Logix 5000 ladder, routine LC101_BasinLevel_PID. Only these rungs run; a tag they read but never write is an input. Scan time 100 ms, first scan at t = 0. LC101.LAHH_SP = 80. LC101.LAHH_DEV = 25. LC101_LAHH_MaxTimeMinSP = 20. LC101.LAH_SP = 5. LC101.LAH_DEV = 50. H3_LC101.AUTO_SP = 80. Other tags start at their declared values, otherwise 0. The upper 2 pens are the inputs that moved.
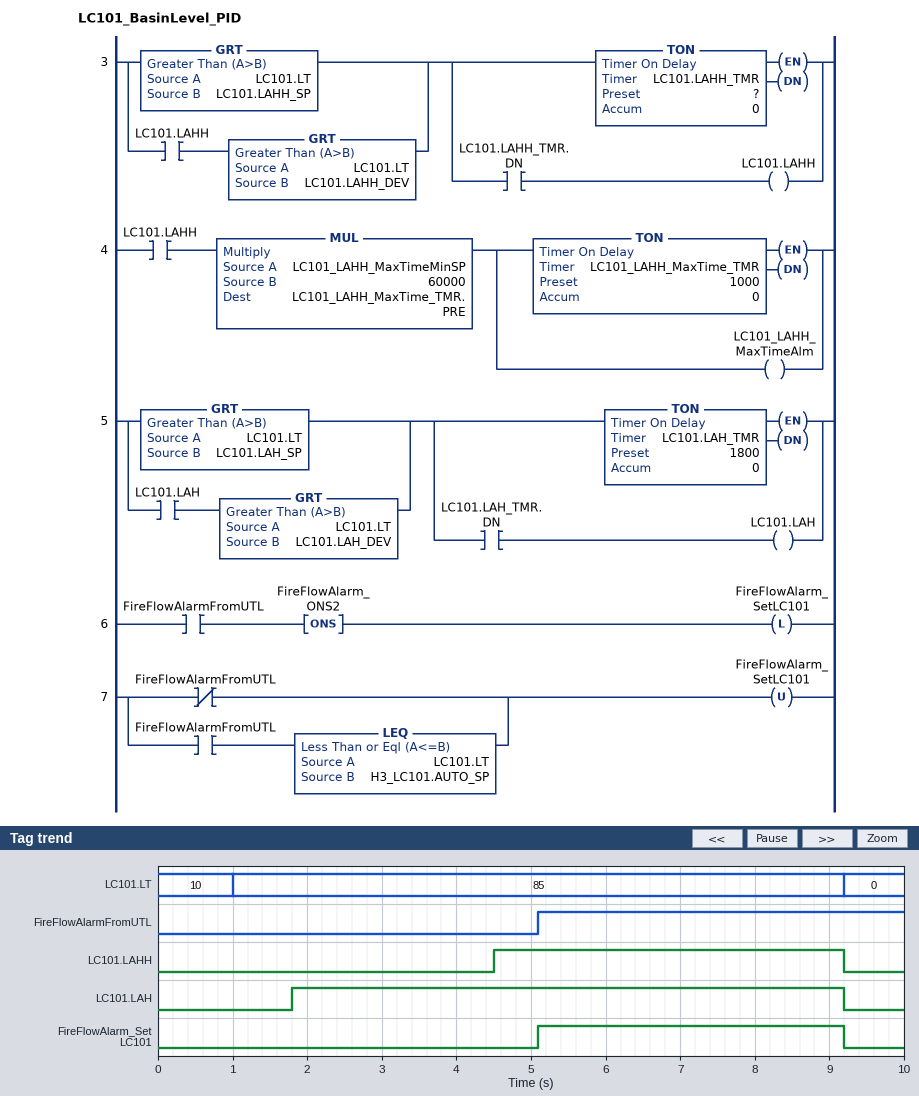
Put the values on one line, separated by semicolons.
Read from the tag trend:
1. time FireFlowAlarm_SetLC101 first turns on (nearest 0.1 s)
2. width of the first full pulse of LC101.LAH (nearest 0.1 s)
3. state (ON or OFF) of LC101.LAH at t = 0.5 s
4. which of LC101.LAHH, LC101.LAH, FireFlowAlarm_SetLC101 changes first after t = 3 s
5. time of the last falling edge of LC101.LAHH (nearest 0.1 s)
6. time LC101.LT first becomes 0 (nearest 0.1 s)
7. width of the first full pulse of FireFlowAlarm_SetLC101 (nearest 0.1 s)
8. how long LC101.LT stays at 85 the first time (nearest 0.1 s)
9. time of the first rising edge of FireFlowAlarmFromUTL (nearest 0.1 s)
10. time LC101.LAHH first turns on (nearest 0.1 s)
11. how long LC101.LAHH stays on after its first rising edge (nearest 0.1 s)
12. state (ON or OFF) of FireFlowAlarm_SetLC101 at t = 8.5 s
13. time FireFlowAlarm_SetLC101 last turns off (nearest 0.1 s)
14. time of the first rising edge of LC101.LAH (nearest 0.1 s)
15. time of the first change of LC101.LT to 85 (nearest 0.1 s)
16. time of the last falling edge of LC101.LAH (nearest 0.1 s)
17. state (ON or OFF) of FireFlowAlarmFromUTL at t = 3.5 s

5.1 s; 7.4 s; OFF; LC101.LAHH; 9.2 s; 9.2 s; 4.1 s; 8.2 s; 5.1 s; 4.5 s; 4.7 s; ON; 9.2 s; 1.8 s; 1.0 s; 9.2 s; OFF
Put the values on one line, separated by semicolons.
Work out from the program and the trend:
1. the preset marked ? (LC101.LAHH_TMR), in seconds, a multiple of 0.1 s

3.5 s
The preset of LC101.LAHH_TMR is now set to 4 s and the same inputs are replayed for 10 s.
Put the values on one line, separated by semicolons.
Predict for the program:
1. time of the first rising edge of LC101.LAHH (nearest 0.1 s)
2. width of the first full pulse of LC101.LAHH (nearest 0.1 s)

5.0 s; 4.2 s
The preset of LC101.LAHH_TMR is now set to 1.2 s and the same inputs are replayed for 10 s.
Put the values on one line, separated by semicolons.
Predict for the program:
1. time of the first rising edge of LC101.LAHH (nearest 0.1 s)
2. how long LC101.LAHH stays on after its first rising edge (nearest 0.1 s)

2.2 s; 7.0 s
